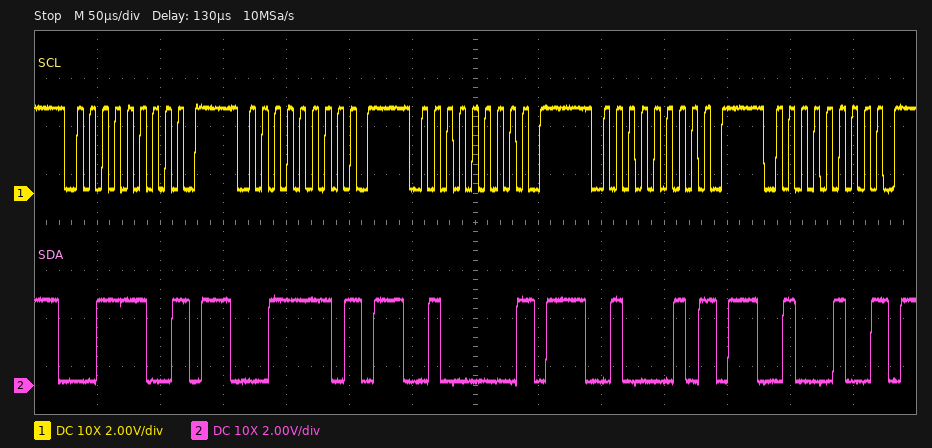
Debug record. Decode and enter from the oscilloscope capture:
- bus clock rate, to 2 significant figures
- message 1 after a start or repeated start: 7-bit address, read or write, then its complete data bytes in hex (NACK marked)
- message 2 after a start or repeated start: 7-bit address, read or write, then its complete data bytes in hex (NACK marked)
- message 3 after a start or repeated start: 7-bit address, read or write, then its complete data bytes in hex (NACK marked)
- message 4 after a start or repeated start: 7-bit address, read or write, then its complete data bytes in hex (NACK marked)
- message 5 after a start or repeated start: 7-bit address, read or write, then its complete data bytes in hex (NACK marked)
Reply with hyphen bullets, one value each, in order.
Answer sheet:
- 100 kHz
- 0x1E write NACK
- 0x1F write NACK
- 0x20 write NACK
- 0x21 write NACK
- 0x22 write NACK
